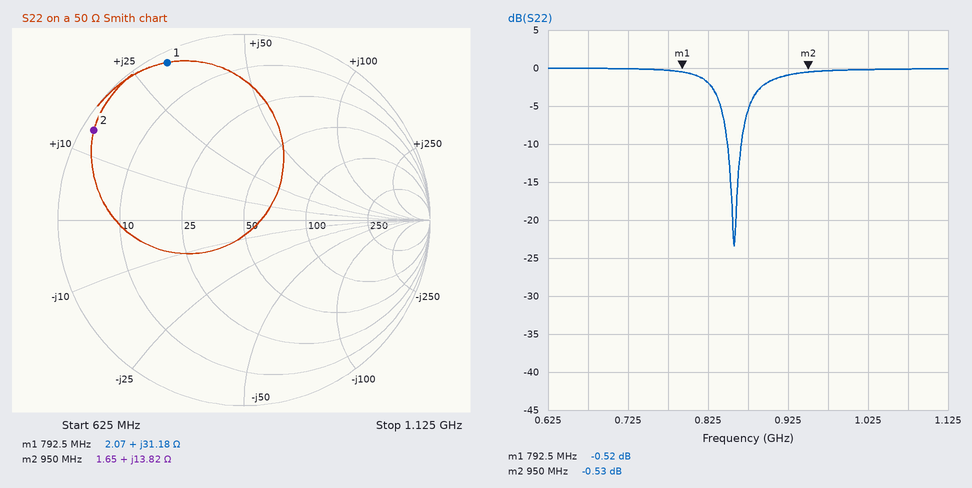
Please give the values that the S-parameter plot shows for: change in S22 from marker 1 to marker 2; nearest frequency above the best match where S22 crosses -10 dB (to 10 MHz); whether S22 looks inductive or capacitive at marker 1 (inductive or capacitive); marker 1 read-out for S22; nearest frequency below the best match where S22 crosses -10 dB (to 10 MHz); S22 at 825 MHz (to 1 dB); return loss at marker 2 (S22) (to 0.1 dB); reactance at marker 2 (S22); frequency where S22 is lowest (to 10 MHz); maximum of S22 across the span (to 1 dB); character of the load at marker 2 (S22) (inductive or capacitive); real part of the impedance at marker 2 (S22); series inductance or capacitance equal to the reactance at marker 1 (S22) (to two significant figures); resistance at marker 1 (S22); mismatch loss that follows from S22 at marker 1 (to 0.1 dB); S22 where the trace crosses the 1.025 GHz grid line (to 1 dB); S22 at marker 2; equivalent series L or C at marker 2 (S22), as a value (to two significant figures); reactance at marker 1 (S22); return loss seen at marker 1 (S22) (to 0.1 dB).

-0.01 dB
870 MHz
inductive
-0.52 dB
850 MHz
-2 dB
0.5 dB
+13.82 Ω
860 MHz
0 dB
inductive
1.65 Ω
6.3 nH
2.07 Ω
9.5 dB
0 dB
-0.53 dB
2.3 nH
+31.18 Ω
0.5 dB
